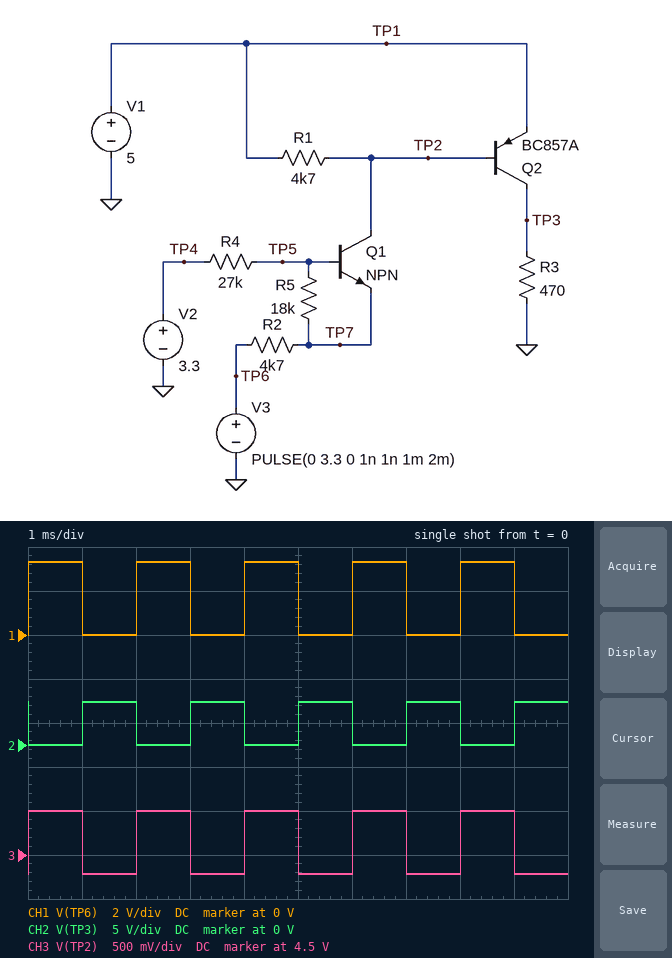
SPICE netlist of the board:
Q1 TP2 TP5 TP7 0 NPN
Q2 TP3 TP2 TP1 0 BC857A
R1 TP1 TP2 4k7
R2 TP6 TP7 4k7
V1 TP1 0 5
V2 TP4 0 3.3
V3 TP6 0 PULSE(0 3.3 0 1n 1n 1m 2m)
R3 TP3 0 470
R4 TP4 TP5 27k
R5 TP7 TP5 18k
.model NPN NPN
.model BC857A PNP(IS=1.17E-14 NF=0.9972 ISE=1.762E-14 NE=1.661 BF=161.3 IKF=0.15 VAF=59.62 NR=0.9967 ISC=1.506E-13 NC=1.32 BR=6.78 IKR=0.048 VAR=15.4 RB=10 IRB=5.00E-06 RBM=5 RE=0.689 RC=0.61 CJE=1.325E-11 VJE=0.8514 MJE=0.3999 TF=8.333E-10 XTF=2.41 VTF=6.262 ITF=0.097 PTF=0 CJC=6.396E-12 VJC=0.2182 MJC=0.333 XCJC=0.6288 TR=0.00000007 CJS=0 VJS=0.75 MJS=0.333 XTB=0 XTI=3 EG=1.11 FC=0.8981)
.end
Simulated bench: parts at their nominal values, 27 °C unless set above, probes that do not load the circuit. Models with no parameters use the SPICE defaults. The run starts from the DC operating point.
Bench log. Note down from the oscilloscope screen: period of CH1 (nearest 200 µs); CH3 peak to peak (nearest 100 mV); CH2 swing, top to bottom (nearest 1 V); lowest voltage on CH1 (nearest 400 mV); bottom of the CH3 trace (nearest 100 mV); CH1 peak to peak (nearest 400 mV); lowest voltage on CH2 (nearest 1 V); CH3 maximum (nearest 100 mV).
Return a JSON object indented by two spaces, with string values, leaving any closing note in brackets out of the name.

{
  "period of CH1": "2.0 ms",
  "CH3 peak to peak": "700 mV",
  "CH2 swing, top to bottom": "5 V",
  "lowest voltage on CH1": "0 V",
  "bottom of the CH3 trace": "4.3 V",
  "CH1 peak to peak": "3.2 V",
  "lowest voltage on CH2": "0 V",
  "CH3 maximum": "5.0 V"
}
